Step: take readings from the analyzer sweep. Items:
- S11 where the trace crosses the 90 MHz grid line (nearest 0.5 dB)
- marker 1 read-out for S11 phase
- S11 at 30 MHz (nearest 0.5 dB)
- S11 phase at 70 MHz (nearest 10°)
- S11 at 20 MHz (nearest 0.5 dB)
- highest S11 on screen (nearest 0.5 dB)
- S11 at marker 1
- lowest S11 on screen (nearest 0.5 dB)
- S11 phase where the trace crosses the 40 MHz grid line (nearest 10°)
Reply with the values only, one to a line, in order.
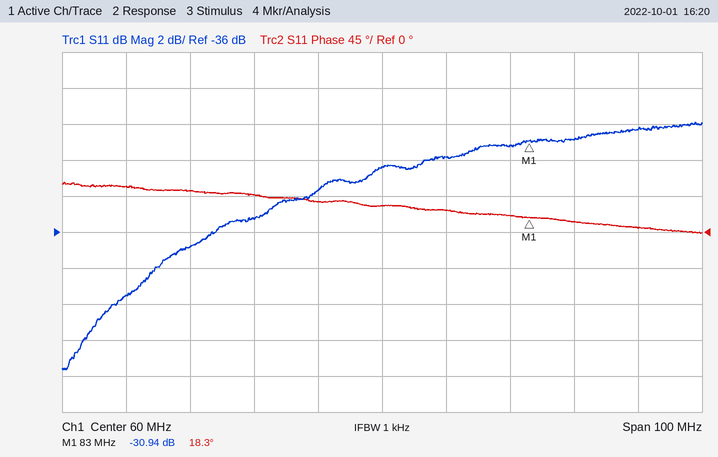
-31.0 dB
18.3°
-37.0 dB
30°
-39.5 dB
-30.0 dB
-30.94 dB
-43.5 dB
50°
